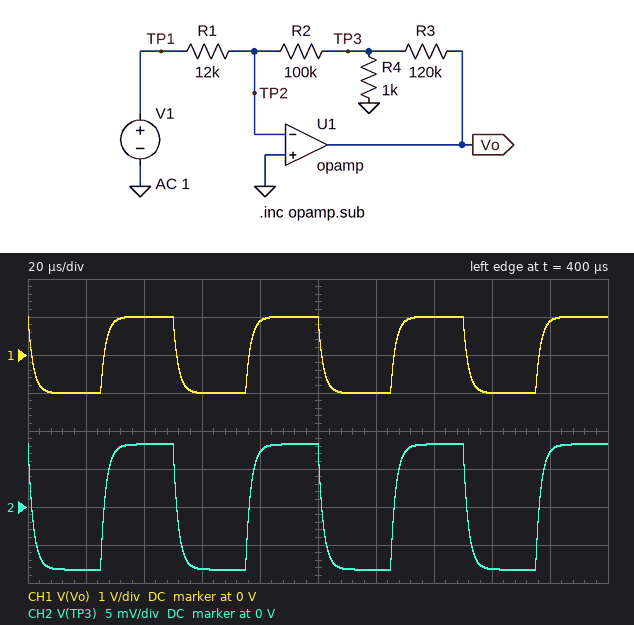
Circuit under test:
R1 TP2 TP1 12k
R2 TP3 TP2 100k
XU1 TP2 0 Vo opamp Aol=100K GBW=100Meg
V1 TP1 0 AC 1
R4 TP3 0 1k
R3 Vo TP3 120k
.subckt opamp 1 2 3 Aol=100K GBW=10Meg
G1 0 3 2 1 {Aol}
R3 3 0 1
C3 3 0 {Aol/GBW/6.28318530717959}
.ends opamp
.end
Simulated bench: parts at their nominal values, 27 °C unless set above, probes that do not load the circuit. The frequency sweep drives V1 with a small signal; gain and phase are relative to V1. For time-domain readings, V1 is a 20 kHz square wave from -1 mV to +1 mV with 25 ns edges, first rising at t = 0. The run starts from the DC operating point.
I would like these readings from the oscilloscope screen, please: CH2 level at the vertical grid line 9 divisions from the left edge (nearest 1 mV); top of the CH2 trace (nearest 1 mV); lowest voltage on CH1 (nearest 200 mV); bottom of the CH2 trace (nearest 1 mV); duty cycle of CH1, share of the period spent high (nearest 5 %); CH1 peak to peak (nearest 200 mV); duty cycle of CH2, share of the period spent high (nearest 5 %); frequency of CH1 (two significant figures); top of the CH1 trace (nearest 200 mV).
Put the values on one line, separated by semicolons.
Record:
7 mV; 8 mV; -1.0 V; -8 mV; 50 %; 2.0 V; 50 %; 20 kHz; 1.0 V
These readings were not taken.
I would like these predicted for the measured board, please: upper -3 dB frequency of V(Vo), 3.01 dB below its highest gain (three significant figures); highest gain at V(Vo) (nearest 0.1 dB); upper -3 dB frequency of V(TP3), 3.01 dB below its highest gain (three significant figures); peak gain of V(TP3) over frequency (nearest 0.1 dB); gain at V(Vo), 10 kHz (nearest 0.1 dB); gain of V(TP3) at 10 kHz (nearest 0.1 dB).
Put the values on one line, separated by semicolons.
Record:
88.8 kHz; 60.1 dB; 88.8 kHz; 18.3 dB; 60.0 dB; 18.3 dB
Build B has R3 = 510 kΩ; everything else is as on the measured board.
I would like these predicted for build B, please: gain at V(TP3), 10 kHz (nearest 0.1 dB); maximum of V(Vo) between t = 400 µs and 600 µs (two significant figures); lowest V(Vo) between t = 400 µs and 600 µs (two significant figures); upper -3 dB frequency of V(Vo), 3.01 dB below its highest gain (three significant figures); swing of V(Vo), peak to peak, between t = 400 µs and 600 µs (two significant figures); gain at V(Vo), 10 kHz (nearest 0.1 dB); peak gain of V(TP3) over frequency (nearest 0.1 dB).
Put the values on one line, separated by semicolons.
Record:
17.2 dB; 3.8 V; -3.8 V; 21.8 kHz; 7.7 V; 71.4 dB; 18.0 dB
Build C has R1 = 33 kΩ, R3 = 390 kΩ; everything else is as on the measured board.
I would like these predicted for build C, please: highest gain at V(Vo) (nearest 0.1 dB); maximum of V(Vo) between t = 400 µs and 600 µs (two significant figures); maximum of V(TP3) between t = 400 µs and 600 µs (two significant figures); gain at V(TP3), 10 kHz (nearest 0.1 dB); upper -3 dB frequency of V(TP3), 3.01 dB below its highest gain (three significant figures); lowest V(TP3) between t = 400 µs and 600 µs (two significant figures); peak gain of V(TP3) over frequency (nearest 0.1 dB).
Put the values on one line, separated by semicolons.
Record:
61.4 dB; 1.2 V; 3.0 mV; 9.4 dB; 64.0 kHz; -3.0 mV; 9.5 dB
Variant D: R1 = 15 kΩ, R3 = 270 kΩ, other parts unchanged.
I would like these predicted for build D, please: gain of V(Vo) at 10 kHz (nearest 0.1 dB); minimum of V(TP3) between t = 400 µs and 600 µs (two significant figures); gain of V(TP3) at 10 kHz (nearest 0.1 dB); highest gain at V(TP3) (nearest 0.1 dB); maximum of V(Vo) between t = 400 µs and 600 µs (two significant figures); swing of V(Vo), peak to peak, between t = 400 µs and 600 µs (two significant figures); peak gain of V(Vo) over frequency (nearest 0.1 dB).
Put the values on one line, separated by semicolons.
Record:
64.9 dB; -6.5 mV; 16.1 dB; 16.3 dB; 1.8 V; 3.6 V; 65.0 dB
